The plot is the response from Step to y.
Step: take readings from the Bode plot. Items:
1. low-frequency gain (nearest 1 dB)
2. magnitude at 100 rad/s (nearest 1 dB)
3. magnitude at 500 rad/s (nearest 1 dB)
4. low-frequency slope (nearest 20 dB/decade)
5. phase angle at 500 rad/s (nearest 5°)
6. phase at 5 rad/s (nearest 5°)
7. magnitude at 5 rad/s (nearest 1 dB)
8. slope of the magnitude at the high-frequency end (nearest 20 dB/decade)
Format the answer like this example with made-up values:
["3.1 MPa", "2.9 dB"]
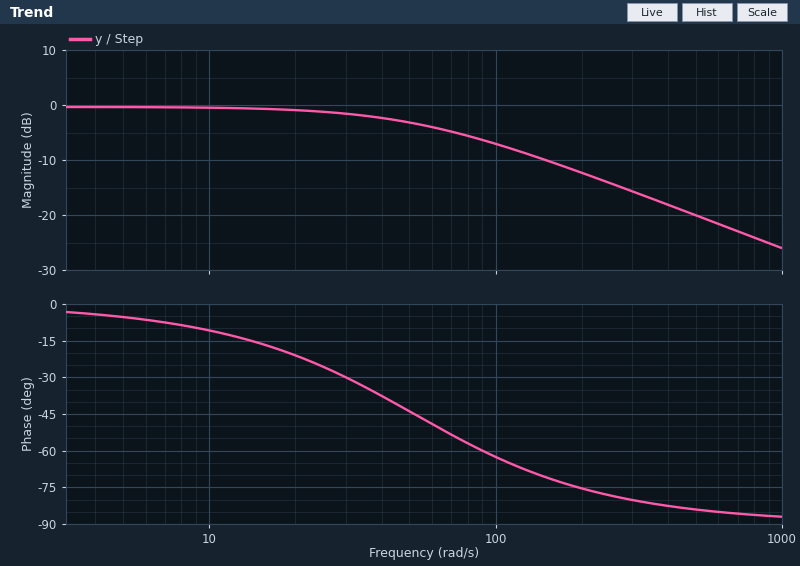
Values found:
["0 dB", "-7 dB", "-20 dB", "0 dB/decade", "-85°", "-5°", "0 dB", "-20 dB/decade"]
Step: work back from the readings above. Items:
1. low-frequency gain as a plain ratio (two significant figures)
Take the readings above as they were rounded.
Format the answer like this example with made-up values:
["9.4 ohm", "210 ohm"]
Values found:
["1.0"]
